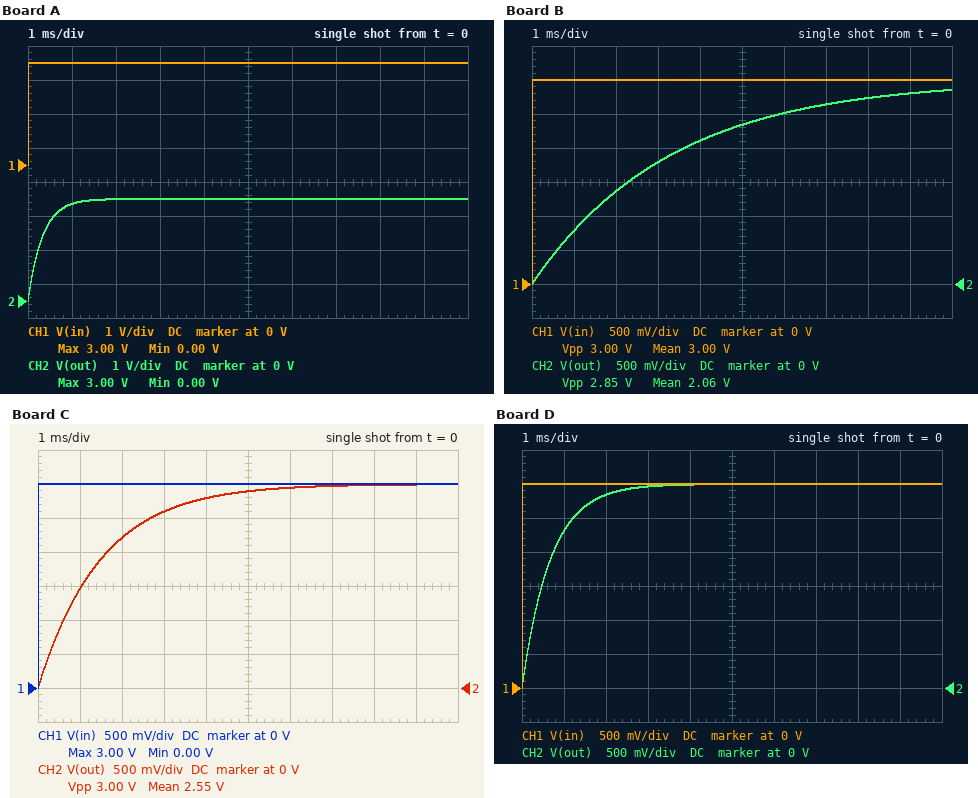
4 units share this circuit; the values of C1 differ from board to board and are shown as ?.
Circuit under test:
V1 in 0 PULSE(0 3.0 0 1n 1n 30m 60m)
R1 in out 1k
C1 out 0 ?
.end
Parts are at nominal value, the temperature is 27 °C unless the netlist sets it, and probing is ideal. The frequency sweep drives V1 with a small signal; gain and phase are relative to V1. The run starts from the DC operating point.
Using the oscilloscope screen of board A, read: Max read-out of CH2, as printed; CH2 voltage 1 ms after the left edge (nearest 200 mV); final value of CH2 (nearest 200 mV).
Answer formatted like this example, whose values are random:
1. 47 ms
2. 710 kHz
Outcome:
1. 3.00 V
2. 2.8 V
3. 3.0 V
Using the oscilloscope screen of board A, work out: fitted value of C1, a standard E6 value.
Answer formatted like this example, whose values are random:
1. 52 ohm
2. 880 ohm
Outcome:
1. 330 nF
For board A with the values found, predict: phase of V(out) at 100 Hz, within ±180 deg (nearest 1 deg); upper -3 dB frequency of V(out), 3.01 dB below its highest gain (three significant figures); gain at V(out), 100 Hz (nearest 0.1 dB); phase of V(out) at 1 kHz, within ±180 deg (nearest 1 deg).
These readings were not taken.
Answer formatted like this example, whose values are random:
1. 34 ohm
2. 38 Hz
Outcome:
1. -12 deg
2. 482 Hz
3. -0.2 dB
4. -64 deg
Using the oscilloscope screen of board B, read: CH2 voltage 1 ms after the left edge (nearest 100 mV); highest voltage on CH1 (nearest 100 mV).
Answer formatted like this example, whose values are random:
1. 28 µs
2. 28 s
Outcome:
1. 800 mV
2. 3.0 V
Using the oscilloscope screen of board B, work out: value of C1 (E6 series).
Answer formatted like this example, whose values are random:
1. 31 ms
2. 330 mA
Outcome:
1. 3.3 µF
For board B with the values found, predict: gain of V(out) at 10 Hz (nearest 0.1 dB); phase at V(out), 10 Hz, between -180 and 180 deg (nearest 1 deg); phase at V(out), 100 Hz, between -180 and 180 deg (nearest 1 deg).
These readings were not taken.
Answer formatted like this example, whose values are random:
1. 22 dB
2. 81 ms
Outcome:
1. -0.2 dB
2. -12 deg
3. -64 deg
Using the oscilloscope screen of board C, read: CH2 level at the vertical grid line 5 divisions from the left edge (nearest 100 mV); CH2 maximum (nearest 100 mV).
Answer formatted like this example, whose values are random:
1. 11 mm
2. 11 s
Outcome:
1. 2.9 V
2. 3.0 V
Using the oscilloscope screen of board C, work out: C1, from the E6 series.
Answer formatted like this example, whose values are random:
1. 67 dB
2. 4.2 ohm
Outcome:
1. 1.5 µF
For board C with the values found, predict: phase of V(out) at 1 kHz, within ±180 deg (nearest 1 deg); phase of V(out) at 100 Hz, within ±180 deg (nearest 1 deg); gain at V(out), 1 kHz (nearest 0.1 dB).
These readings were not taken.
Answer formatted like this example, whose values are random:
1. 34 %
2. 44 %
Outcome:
1. -84 deg
2. -43 deg
3. -19.5 dB
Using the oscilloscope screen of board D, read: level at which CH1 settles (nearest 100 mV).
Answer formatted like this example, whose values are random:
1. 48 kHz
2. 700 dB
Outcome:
1. 3.0 V
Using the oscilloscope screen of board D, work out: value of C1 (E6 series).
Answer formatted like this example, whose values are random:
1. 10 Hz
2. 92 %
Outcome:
1. 680 nF
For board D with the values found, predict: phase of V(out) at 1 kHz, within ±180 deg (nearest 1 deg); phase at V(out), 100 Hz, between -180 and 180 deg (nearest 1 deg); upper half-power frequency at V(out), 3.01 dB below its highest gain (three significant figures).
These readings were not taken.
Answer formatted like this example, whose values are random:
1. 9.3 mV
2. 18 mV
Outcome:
1. -77 deg
2. -23 deg
3. 234 Hz
